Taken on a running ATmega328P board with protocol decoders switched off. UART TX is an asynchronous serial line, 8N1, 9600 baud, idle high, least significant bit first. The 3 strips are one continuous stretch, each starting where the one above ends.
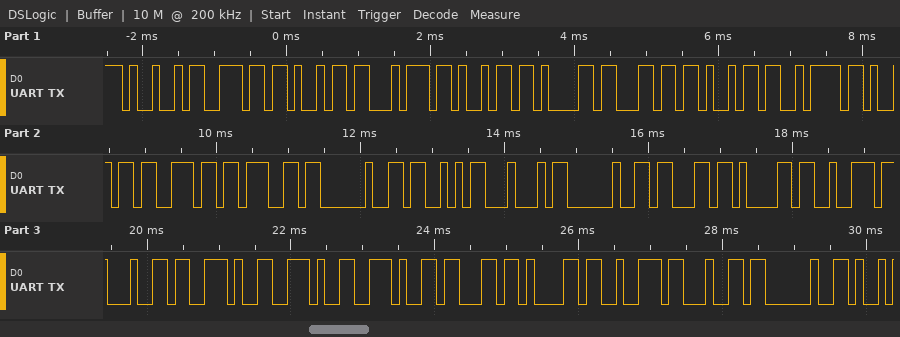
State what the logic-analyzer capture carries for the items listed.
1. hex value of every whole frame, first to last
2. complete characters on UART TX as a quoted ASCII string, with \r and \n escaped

49 6E 69 74 69 61 6C 69 7A 69 6E 67 20 53 44 20 63 61 72 64 2E 2E 2E 63 61 72 64 20
"Initializing SD card...card "
